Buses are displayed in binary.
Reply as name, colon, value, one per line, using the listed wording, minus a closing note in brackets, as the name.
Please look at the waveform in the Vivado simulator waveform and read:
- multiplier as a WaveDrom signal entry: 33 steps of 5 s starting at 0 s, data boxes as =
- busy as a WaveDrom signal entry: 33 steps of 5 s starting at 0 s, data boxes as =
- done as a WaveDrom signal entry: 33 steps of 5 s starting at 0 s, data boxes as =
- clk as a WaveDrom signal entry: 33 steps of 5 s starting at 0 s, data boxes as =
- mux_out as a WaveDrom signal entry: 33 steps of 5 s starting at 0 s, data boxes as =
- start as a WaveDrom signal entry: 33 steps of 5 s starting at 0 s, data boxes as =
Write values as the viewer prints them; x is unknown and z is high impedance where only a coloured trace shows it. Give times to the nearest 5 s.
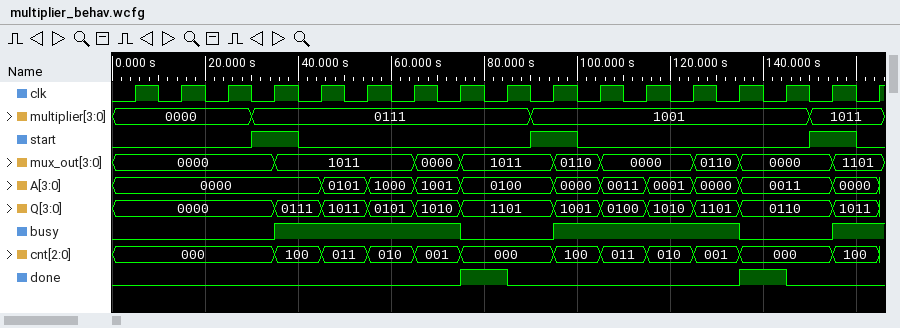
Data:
multiplier as a WaveDrom signal entry: 33 steps of 5 s starting at 0 s, data boxes as =: {name: 'multiplier', wave: '=.....=...........=...........=..', data: '0000 0111 1001 1011'}
busy as a WaveDrom signal entry: 33 steps of 5 s starting at 0 s, data boxes as =: {name: 'busy', wave: '0......1.......0...1.......0...1.'}
done as a WaveDrom signal entry: 33 steps of 5 s starting at 0 s, data boxes as =: {name: 'done', wave: '0..............1.0.........1.0...'}
clk as a WaveDrom signal entry: 33 steps of 5 s starting at 0 s, data boxes as =: {name: 'clk', wave: '010101010101010101010101010101010'}
mux_out as a WaveDrom signal entry: 33 steps of 5 s starting at 0 s, data boxes as =: {name: 'mux_out', wave: '=......=.....=.=...=.=...=.=...=.', data: '0000 1011 0000 1011 0110 0000 0110 0000 1101'}
start as a WaveDrom signal entry: 33 steps of 5 s starting at 0 s, data boxes as =: {name: 'start', wave: '0.....1.0.........1.0.........1.0'}
